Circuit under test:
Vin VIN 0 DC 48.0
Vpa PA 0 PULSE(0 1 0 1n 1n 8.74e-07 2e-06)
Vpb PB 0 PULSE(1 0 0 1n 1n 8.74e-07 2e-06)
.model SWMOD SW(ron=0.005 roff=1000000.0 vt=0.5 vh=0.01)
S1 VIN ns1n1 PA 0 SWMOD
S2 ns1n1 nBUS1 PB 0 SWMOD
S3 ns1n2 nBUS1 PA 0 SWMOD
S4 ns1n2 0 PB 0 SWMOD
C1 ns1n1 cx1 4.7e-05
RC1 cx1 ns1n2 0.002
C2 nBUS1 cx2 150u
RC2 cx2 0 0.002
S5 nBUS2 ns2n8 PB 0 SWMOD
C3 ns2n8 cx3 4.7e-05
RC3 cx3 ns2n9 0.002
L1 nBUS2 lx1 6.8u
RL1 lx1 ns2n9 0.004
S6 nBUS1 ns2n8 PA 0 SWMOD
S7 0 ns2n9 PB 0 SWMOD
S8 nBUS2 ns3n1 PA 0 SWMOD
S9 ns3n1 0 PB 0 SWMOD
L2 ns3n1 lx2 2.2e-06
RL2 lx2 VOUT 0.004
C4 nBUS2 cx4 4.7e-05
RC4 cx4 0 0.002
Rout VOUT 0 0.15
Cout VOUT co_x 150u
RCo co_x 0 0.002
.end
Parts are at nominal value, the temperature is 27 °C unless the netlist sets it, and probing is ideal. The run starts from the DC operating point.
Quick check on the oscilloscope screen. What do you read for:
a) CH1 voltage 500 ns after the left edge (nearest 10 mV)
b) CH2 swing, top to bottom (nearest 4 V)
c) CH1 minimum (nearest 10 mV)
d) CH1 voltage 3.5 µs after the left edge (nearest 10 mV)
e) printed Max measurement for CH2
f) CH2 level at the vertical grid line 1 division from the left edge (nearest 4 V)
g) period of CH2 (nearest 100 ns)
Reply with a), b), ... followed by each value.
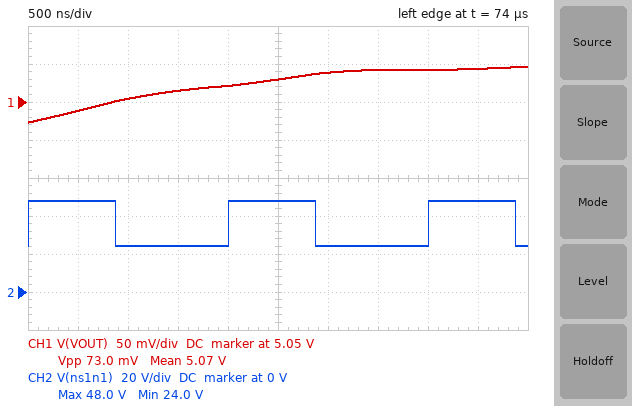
a) 5.04 V
b) 24 V
c) 5.02 V
d) 5.09 V
e) 48.0 V
f) 48 V
g) 2.0 µs
